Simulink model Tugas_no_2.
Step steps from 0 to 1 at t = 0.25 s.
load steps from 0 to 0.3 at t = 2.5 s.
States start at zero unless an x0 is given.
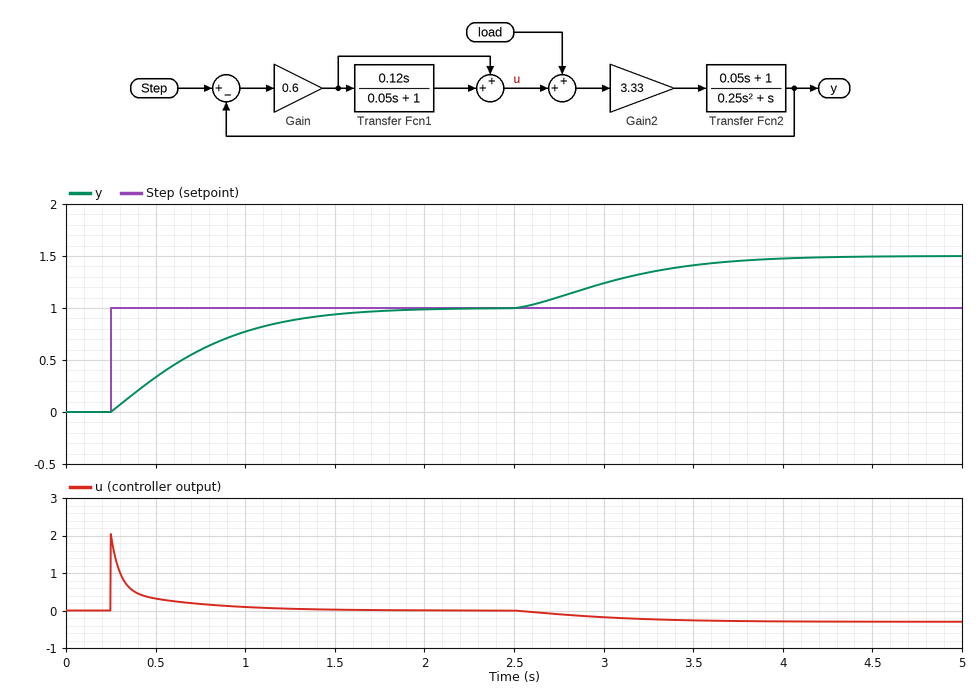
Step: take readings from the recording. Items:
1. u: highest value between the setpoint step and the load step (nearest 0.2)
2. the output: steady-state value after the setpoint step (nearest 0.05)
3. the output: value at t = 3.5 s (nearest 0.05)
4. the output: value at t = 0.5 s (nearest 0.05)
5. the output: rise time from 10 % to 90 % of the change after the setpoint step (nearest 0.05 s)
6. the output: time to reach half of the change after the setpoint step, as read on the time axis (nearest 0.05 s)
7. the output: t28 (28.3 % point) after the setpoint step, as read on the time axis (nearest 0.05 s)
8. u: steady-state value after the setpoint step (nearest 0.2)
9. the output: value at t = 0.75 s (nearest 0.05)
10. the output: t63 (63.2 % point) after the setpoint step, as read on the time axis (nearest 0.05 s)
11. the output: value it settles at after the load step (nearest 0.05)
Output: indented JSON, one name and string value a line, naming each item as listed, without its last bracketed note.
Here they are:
{
  "u: highest value between the setpoint step and the load step": "2.0",
  "the output: steady-state value after the setpoint step": "1.00",
  "the output: value at t = 3.5 s": "1.40",
  "the output: value at t = 0.5 s": "0.35",
  "the output: rise time from 10 % to 90 % of the change after the setpoint step": "1.00 s",
  "the output: time to reach half of the change after the setpoint step, as read on the time axis": "0.65 s",
  "the output: t28 (28.3 % point) after the setpoint step, as read on the time axis": "0.45 s",
  "u: steady-state value after the setpoint step": "0.0",
  "the output: value at t = 0.75 s": "0.60",
  "the output: t63 (63.2 % point) after the setpoint step, as read on the time axis": "0.80 s",
  "the output: value it settles at after the load step": "1.50"
}
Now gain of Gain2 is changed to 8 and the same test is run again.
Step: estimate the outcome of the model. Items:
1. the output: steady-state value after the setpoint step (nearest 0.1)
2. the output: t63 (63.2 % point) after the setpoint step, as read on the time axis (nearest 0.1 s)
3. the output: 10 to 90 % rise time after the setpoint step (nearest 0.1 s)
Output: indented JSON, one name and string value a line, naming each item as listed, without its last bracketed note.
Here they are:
{
  "the output: steady-state value after the setpoint step": "1.0",
  "the output: t63 (63.2 % point) after the setpoint step, as read on the time axis": "0.5 s",
  "the output: 10 to 90 % rise time after the setpoint step": "0.4 s"
}
